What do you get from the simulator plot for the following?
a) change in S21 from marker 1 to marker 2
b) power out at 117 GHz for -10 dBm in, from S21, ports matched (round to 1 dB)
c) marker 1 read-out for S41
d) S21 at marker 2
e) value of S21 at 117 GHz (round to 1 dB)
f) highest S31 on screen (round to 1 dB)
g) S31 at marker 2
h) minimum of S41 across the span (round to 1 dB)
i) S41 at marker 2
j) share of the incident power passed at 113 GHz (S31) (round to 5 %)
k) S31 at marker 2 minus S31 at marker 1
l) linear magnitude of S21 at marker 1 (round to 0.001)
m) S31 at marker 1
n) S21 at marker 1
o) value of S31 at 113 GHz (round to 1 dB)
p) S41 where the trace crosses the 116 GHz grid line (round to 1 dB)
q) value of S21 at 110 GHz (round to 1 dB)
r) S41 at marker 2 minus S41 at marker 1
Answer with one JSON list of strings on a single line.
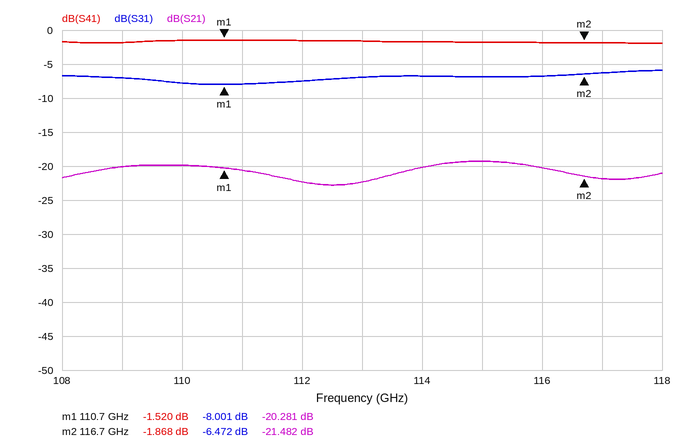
["-1.201 dB", "-32 dBm", "-1.520 dB", "-21.482 dB", "-22 dB", "-6 dB", "-6.472 dB", "-2 dB", "-1.868 dB", "20 %", "1.529 dB", "0.097", "-8.001 dB", "-20.281 dB", "-7 dB", "-2 dB", "-20 dB", "-0.348 dB"]
